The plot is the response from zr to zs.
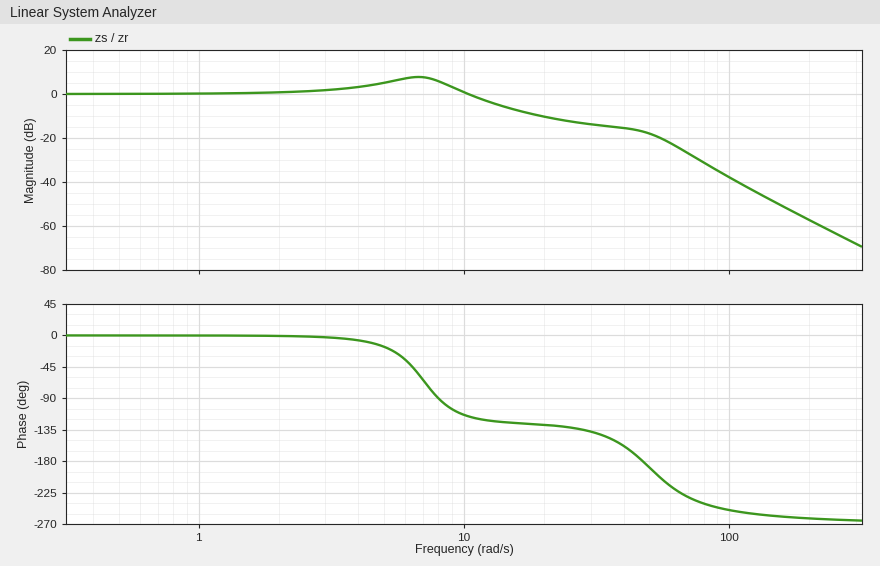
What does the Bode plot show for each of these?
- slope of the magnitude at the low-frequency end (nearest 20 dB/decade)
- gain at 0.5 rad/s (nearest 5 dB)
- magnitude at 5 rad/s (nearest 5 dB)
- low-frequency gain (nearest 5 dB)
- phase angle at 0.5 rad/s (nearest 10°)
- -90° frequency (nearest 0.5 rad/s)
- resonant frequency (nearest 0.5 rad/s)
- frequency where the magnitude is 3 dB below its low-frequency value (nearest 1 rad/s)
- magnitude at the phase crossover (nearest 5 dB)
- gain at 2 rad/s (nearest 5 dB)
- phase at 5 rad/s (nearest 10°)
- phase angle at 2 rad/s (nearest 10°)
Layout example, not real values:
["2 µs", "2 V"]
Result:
["0 dB/decade", "0 dB", "5 dB", "0 dB", "0°", "8.0 rad/s", "6.5 rad/s", "12 rad/s", "-15 dB", "0 dB", "-20°", "0°"]
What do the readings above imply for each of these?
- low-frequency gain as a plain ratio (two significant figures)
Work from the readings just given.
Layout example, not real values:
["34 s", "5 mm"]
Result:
["1.0"]
